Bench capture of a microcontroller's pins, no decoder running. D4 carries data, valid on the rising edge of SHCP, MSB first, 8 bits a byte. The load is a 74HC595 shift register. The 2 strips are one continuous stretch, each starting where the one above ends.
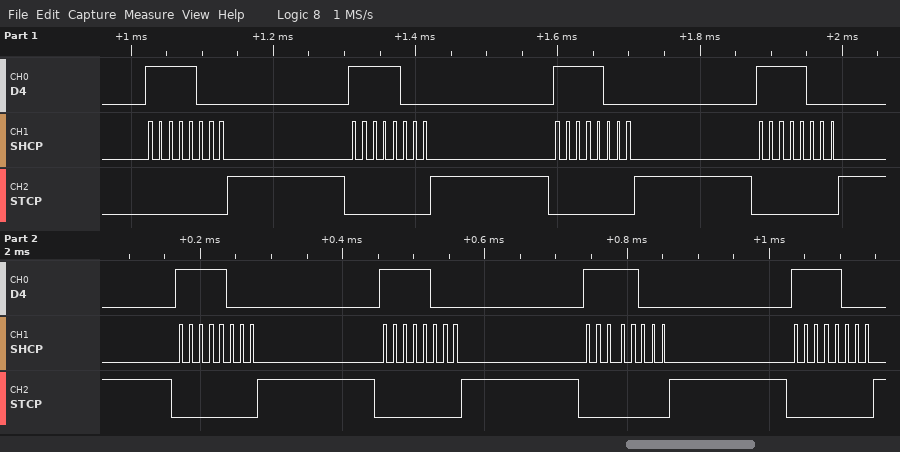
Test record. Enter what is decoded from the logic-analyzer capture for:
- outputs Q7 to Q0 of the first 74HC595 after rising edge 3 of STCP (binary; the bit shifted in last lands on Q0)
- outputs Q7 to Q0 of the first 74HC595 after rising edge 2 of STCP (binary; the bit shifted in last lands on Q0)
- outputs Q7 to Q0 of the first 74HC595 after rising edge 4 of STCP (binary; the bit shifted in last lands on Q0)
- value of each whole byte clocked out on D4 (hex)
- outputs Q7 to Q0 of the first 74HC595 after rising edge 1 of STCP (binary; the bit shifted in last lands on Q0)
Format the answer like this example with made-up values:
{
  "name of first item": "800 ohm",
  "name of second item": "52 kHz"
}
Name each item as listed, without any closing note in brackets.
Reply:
{
  "outputs Q7 to Q0 of the first 74HC595 after rising edge 3 of STCP": "11111000",
  "outputs Q7 to Q0 of the first 74HC595 after rising edge 2 of STCP": "11111000",
  "outputs Q7 to Q0 of the first 74HC595 after rising edge 4 of STCP": "11111000",
  "value of each whole byte clocked out on D4": "F8 F8 F8 F8 F8 F8 F8 F8",
  "outputs Q7 to Q0 of the first 74HC595 after rising edge 1 of STCP": "11111000"
}
